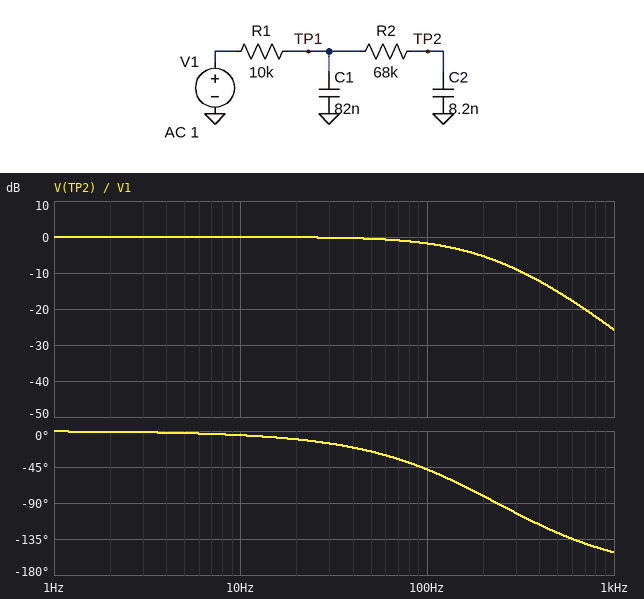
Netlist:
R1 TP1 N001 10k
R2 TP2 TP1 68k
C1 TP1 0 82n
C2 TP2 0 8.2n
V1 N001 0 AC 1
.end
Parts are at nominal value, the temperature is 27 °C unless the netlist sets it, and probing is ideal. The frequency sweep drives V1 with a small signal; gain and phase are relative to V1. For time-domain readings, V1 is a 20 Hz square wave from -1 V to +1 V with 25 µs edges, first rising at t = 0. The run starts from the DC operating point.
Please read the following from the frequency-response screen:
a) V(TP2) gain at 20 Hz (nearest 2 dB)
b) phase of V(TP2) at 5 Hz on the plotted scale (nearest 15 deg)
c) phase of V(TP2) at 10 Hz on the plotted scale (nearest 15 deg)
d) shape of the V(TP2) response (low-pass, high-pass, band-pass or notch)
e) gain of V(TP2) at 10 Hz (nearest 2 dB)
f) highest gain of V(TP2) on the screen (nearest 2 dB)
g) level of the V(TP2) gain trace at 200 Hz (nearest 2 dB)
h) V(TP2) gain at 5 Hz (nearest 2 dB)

0 dB
0 deg
0 deg
low-pass
0 dB
0 dB
-6 dB
0 dB
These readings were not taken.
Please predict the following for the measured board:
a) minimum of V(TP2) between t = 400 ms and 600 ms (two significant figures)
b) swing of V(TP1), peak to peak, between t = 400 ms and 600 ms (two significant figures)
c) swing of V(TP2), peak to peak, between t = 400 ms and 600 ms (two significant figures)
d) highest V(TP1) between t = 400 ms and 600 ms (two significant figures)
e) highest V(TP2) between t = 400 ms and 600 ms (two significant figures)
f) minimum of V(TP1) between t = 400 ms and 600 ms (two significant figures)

-1.0 V
2.0 V
2.0 V
1.0 V
1.0 V
-1.0 V
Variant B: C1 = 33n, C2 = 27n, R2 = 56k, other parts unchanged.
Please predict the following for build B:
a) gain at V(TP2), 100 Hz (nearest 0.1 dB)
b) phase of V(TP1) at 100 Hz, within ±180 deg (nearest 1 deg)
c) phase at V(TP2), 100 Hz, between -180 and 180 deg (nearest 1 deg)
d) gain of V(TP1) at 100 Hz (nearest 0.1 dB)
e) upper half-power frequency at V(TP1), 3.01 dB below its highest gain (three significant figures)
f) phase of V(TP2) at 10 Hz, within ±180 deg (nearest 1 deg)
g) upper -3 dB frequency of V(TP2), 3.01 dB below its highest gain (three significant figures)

-3.8 dB
-15 deg
-59 deg
-1.0 dB
364 Hz
-8 deg
84.7 Hz
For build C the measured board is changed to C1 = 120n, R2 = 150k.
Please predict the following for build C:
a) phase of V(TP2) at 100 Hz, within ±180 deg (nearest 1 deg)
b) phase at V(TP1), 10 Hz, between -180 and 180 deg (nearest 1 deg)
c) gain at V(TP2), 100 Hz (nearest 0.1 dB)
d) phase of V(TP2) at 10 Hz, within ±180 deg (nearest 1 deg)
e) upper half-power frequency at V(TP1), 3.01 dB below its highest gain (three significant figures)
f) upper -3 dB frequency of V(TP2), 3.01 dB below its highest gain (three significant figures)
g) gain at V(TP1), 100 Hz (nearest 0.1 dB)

-75 deg
-5 deg
-4.3 dB
-9 deg
124 Hz
80.4 Hz
-2.2 dB
